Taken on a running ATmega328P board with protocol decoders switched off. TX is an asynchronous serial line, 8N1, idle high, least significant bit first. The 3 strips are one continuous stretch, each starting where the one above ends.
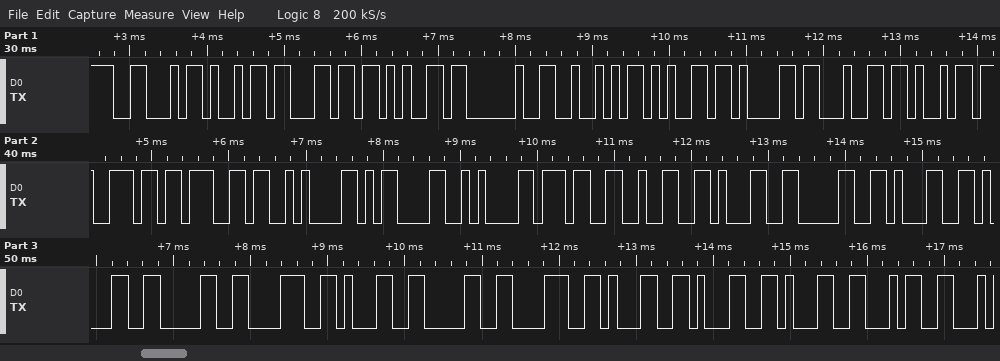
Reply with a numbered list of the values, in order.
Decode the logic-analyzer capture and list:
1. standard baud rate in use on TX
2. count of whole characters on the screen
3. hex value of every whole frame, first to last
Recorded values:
1. 9600 baud
2. 30
3. 46 69 6C 65 20 52 65 61 64 69 6E 67 0A 0D 0A 37 32 31 30 31 31 30 38 31 30 38 31 31 31 34
